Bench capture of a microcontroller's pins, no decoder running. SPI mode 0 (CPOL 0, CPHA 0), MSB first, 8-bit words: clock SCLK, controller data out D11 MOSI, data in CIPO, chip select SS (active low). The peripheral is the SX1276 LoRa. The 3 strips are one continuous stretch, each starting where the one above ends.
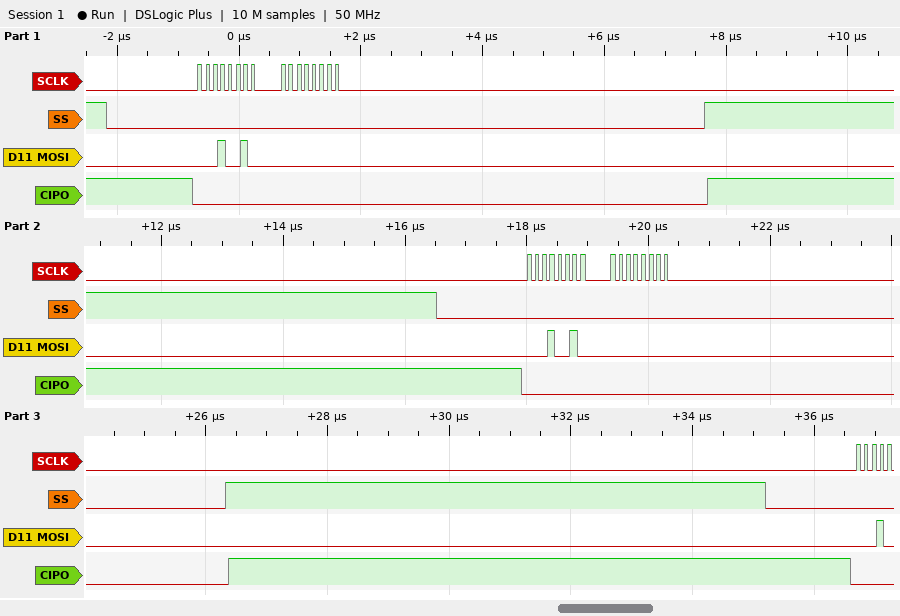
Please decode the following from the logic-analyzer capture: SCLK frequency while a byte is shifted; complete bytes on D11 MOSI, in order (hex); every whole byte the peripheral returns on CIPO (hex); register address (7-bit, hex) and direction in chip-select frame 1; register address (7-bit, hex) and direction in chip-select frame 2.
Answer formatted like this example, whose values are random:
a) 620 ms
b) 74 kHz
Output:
a) 8 MHz
b) 0x12 0x00 0x12 0x00
c) 0x00 0x00 0x00 0x00
d) 0x12 read
e) 0x12 read
